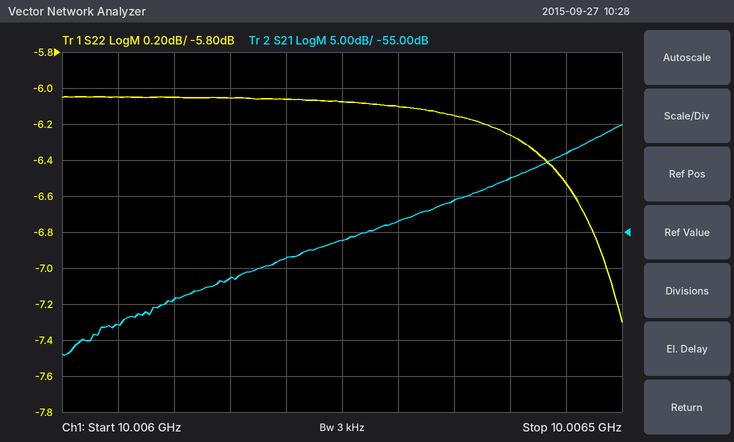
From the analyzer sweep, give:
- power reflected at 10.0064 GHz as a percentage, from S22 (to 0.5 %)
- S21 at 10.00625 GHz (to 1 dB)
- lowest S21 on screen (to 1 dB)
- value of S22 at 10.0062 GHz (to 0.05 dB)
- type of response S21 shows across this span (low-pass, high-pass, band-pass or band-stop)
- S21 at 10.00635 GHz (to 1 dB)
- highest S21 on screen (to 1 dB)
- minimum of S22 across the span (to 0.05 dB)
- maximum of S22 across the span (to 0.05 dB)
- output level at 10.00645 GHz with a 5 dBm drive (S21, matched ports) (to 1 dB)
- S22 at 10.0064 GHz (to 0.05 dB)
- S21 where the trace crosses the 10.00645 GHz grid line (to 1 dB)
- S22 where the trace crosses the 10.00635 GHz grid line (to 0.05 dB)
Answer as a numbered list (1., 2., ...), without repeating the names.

1. 23.5 %
2. -56 dB
3. -72 dB
4. -6.05 dB
5. high-pass
6. -51 dB
7. -40 dB
8. -7.30 dB
9. -6.05 dB
10. -39 dBm
11. -6.25 dB
12. -44 dB
13. -6.15 dB
